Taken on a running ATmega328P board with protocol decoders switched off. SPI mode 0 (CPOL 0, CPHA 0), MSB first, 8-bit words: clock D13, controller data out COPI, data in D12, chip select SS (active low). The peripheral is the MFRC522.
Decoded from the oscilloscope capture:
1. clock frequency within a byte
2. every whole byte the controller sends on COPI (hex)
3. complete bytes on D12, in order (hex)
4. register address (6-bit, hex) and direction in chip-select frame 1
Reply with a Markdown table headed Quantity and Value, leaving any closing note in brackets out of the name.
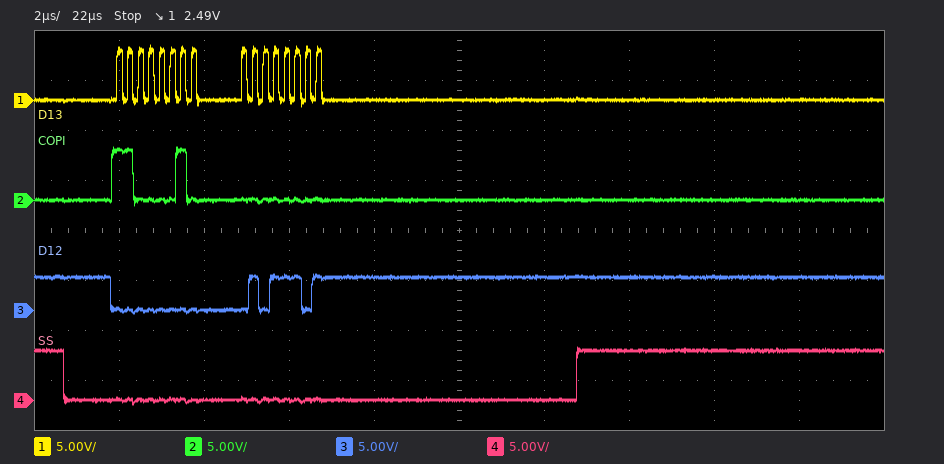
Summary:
| Quantity | Value |
|---|---|
| clock frequency within a byte | 4 MHz |
| every whole byte the controller sends on COPI | C2 00 |
| complete bytes on D12, in order | 00 5D |
| register address (6-bit, hex) and direction in chip-select frame 1 | 0x21 read |
